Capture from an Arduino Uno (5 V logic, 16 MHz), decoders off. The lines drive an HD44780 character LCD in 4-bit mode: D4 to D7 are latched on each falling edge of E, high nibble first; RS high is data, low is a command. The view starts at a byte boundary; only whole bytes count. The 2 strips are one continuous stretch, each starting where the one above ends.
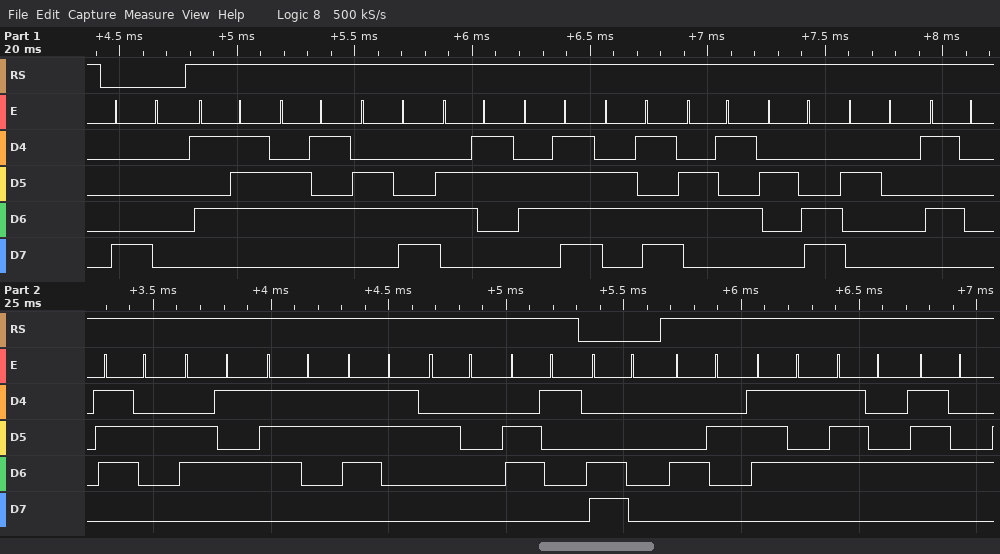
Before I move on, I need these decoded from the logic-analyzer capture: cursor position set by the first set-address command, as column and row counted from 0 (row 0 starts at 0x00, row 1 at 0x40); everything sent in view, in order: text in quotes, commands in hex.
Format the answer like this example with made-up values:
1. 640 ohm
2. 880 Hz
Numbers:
1. column 0, row 0
2. 0x80 "Welcome, Press a" 0xC0 "Butt"
